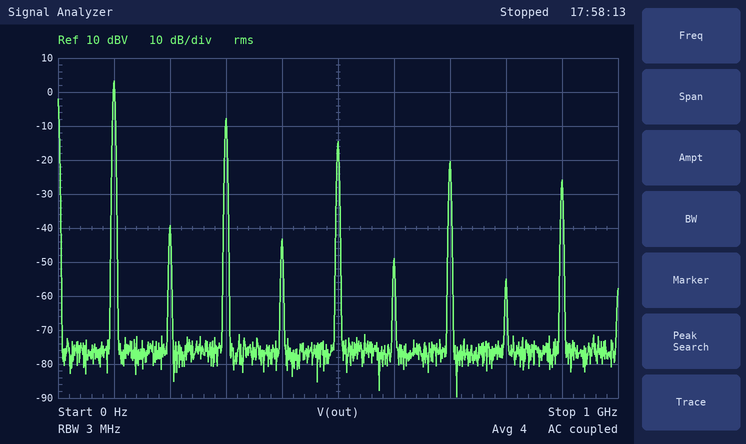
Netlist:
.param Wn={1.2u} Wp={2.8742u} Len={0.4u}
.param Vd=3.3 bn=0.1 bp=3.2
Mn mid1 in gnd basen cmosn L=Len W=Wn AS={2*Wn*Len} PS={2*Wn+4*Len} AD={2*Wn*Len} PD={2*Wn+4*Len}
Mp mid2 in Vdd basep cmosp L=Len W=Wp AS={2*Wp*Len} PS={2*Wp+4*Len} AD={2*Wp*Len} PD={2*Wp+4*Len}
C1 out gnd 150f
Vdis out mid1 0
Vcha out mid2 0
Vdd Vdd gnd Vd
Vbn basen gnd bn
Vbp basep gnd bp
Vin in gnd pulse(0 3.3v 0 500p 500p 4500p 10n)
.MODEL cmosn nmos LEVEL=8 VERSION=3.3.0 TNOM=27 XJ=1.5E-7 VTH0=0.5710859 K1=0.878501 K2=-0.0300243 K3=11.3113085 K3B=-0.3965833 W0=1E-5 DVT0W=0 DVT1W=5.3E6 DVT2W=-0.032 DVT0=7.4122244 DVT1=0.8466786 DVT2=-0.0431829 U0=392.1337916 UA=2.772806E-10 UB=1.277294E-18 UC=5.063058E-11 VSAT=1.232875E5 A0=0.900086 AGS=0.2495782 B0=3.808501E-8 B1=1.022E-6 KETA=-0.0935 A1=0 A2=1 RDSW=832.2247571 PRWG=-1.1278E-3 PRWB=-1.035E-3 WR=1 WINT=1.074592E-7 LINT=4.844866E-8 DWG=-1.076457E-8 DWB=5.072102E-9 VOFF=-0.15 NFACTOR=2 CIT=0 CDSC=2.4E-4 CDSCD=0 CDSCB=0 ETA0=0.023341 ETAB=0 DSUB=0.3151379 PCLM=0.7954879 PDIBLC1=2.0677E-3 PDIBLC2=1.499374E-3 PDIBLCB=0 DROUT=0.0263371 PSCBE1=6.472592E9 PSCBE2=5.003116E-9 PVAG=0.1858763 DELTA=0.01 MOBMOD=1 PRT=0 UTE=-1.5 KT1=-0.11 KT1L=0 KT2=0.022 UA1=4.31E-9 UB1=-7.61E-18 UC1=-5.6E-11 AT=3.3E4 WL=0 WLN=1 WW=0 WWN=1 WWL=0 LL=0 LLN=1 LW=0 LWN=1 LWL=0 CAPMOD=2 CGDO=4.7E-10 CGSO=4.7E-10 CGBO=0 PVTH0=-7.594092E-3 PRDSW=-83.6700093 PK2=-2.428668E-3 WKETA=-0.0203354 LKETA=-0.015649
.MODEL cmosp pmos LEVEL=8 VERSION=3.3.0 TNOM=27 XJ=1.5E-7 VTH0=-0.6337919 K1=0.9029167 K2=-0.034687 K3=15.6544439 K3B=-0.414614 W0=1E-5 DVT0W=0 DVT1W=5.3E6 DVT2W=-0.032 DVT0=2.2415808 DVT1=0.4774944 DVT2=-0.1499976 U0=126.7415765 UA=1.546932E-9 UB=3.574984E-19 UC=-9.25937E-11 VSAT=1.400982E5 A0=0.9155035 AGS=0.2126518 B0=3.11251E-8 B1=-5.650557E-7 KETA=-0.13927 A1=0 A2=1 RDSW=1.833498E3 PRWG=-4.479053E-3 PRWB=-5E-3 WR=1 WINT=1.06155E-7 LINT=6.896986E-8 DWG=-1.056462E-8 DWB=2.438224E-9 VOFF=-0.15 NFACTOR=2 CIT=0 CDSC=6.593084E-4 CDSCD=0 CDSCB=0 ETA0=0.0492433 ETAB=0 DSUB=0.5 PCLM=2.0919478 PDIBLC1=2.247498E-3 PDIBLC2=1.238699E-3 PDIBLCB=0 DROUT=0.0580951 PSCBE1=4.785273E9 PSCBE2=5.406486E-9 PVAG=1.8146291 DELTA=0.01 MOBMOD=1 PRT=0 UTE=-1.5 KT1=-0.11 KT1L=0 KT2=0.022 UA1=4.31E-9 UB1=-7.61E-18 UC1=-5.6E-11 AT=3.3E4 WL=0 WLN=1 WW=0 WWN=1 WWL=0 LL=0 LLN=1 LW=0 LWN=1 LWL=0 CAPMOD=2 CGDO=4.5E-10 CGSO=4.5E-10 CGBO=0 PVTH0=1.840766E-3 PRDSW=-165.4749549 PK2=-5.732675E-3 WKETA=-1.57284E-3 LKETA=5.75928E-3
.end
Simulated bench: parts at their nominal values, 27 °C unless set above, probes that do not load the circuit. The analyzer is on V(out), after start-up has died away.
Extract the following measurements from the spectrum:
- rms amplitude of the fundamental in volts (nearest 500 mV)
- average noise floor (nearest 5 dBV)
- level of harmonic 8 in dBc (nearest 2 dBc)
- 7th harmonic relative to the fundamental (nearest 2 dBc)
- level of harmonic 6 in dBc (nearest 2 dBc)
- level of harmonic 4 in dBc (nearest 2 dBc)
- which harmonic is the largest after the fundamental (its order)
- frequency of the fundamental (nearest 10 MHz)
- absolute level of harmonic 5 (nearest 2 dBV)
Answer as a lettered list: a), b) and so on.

a) 1.5 V
b) -75 dBV
c) -58 dBc
d) -24 dBc
e) -52 dBc
f) -46 dBc
g) 3
h) 100 MHz
i) -14 dBV
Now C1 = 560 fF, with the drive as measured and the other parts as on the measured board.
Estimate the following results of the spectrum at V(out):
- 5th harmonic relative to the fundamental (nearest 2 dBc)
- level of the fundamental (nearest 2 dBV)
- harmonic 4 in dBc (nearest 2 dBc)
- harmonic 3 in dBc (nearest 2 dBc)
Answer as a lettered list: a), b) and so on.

a) -30 dBc
b) 2 dBV
c) -60 dBc
d) -20 dBc
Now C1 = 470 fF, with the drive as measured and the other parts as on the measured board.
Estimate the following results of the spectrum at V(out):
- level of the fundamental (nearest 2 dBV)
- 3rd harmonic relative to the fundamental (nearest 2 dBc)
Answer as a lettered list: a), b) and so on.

a) 2 dBV
b) -18 dBc
